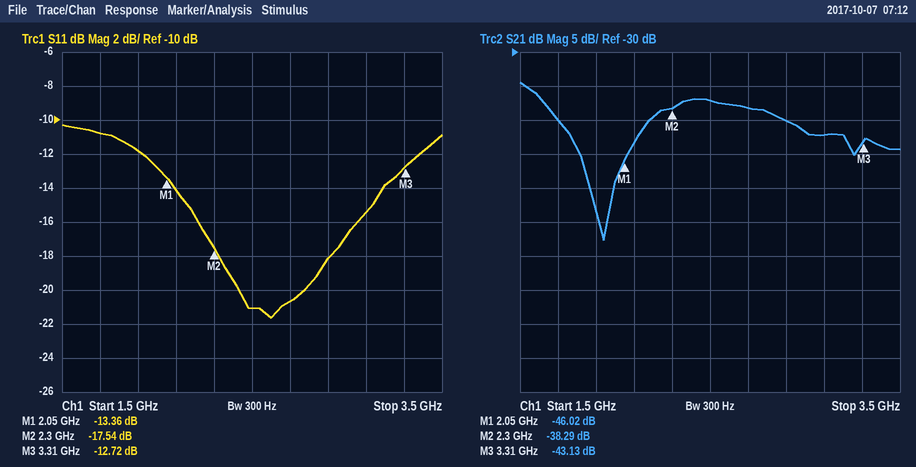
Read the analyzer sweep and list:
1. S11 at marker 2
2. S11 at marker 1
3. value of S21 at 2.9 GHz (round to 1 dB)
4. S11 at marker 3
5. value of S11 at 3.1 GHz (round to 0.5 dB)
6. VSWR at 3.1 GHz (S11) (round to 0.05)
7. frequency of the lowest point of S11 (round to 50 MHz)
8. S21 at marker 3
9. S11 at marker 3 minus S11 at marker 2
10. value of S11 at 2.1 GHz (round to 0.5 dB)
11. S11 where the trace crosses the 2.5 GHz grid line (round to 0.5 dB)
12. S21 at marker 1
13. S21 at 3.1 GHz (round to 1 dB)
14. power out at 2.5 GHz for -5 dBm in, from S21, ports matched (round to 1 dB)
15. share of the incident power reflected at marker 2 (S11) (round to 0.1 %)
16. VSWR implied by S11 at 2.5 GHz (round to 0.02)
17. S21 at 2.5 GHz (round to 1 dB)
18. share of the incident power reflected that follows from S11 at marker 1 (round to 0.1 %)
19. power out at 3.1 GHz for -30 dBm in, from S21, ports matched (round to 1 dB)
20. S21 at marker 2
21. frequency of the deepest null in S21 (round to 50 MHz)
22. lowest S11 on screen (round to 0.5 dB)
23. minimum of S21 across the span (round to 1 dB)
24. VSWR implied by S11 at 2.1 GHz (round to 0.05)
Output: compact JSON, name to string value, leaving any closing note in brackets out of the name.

{"S11 at marker 2": "-17.54 dB", "S11 at marker 1": "-13.36 dB", "value of S21 at 2.9 GHz": "-40 dB", "S11 at marker 3": "-12.72 dB", "value of S11 at 3.1 GHz": "-15.5 dB", "VSWR at 3.1 GHz (S11)": "1.40", "frequency of the lowest point of S11": "2.60 GHz", "S21 at marker 3": "-43.13 dB", "S11 at marker 3 minus S11 at marker 2": "4.82 dB", "value of S11 at 2.1 GHz": "-14.0 dB", "S11 where the trace crosses the 2.5 GHz grid line": "-21.0 dB", "S21 at marker 1": "-46.02 dB", "S21 at 3.1 GHz": "-42 dB", "power out at 2.5 GHz for -5 dBm in, from S21, ports matched": "-42 dBm", "share of the incident power reflected at marker 2 (S11)": "1.8 %", "VSWR implied by S11 at 2.5 GHz": "1.20", "S21 at 2.5 GHz": "-37 dB", "share of the incident power reflected that follows from S11 at marker 1": "4.6 %", "power out at 3.1 GHz for -30 dBm in, from S21, ports matched": "-72 dBm", "S21 at marker 2": "-38.29 dB", "frequency of the deepest null in S21": "1.95 GHz", "lowest S11 on screen": "-21.5 dB", "minimum of S21 across the span": "-58 dB", "VSWR implied by S11 at 2.1 GHz": "1.50"}
